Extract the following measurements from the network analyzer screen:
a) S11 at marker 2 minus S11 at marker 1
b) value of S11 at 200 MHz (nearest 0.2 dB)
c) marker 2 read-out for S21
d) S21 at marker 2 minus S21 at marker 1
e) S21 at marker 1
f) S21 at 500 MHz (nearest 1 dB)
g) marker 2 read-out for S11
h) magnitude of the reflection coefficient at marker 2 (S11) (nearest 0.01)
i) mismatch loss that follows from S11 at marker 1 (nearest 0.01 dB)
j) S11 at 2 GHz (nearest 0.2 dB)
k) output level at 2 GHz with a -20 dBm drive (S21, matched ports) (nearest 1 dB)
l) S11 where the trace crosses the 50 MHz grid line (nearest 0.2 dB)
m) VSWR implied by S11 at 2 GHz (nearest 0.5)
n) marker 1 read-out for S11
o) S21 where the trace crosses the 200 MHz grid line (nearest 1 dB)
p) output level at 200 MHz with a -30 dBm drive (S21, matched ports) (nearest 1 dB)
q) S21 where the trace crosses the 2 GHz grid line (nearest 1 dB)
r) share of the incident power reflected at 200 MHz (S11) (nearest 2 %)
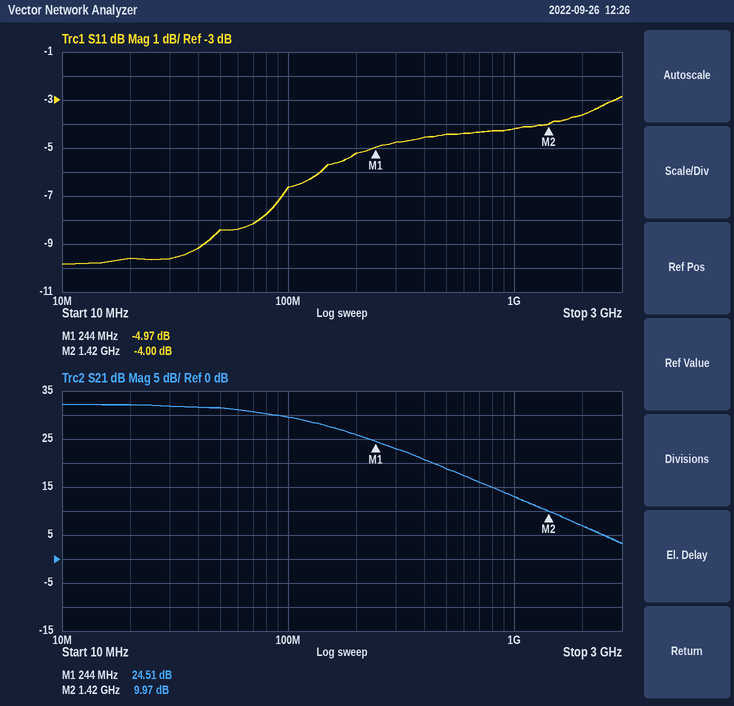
0.97 dB
-5.2 dB
9.97 dB
-14.54 dB
24.51 dB
19 dB
-4.00 dB
0.63
1.66 dB
-3.6 dB
-13 dBm
-8.4 dB
5.0
-4.97 dB
26 dB
-4 dBm
7 dB
30 %
